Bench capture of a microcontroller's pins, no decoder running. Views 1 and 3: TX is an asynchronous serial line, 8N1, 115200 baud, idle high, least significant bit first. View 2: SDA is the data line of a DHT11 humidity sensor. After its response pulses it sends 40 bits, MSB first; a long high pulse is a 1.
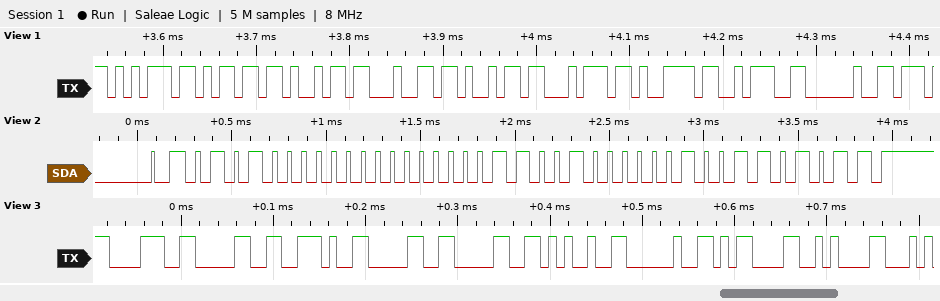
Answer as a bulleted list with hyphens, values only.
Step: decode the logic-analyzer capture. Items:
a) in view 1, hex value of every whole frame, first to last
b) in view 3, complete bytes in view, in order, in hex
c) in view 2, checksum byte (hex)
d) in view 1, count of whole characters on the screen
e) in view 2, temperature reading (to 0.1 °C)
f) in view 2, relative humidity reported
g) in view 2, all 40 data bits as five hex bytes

- 75 6D 69 64 69 74 79 3A 20
- 38 30 2E 30 30 25 20 0D 0A
- 0x6B
- 9
- 25.2 °C
- 80 %
- 50 00 19 02 6B
